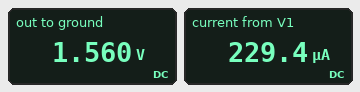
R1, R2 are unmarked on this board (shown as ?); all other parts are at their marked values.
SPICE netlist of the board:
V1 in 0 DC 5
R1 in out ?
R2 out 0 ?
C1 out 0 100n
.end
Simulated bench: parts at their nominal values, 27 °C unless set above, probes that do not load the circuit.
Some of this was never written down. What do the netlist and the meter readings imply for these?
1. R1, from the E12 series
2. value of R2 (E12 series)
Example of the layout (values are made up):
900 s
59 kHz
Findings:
15 kΩ
6.8 kΩ
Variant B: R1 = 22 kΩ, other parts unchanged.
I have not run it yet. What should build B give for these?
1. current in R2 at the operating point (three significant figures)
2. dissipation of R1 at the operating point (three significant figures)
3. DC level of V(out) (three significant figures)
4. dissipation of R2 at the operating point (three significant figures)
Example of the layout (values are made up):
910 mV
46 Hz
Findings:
174 µA
663 µW
1.18 V
205 µW
